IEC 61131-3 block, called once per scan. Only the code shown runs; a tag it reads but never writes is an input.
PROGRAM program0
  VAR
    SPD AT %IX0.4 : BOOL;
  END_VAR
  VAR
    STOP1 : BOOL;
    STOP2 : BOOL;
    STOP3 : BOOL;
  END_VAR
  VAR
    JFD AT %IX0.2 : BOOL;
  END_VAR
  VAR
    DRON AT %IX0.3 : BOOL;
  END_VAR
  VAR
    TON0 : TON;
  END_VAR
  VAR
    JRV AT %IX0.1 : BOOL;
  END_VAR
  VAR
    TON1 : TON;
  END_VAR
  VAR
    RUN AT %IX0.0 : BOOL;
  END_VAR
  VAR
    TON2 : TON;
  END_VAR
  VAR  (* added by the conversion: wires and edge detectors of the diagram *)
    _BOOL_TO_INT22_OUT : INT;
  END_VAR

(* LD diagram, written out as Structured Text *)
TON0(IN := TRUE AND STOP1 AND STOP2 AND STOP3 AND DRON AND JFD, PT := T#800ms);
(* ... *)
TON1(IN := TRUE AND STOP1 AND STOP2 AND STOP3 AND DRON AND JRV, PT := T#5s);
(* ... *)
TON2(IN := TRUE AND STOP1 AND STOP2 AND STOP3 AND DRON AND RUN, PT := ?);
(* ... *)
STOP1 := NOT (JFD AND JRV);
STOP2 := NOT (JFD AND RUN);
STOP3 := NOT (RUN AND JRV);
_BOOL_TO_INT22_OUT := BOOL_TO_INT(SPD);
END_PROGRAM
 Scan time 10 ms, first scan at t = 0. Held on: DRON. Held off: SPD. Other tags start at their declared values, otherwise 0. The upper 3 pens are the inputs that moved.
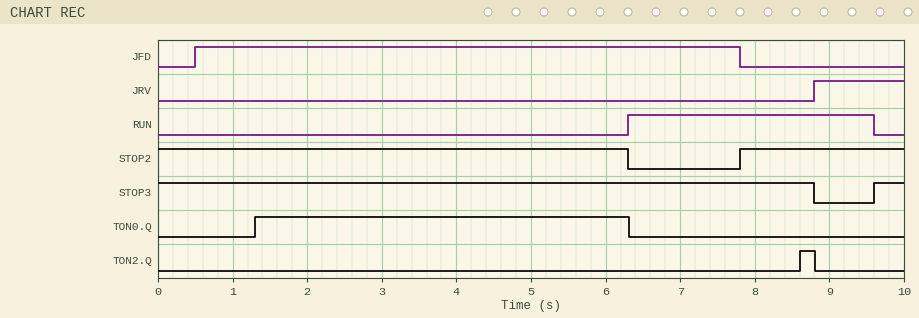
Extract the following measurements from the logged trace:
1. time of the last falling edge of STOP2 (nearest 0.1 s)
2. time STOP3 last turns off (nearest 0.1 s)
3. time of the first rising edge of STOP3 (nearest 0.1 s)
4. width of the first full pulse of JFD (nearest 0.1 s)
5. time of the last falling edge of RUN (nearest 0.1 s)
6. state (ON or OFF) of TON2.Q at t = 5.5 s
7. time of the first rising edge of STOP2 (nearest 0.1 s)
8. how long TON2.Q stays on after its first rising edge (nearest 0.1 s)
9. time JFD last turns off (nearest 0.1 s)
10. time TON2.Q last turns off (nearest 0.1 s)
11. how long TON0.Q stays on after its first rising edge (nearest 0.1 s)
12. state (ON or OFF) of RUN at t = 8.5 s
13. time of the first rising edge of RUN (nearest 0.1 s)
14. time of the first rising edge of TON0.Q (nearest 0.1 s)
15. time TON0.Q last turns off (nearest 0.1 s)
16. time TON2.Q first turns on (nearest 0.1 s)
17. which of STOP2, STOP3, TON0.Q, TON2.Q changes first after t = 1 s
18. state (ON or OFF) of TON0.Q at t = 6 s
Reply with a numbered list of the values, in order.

1. 6.3 s
2. 8.8 s
3. 9.6 s
4. 7.3 s
5. 9.6 s
6. OFF
7. 7.8 s
8. 0.2 s
9. 7.8 s
10. 8.8 s
11. 5.0 s
12. ON
13. 6.3 s
14. 1.3 s
15. 6.3 s
16. 8.6 s
17. TON0.Q
18. ON
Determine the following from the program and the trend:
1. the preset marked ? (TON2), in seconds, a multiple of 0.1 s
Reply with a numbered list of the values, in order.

1. 0.8 s
